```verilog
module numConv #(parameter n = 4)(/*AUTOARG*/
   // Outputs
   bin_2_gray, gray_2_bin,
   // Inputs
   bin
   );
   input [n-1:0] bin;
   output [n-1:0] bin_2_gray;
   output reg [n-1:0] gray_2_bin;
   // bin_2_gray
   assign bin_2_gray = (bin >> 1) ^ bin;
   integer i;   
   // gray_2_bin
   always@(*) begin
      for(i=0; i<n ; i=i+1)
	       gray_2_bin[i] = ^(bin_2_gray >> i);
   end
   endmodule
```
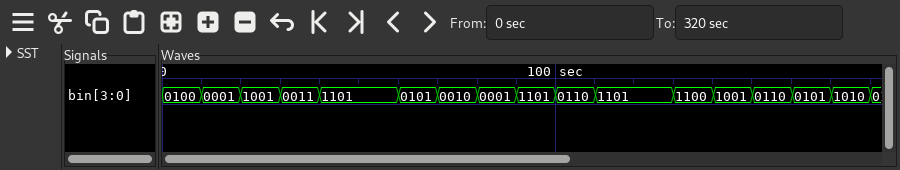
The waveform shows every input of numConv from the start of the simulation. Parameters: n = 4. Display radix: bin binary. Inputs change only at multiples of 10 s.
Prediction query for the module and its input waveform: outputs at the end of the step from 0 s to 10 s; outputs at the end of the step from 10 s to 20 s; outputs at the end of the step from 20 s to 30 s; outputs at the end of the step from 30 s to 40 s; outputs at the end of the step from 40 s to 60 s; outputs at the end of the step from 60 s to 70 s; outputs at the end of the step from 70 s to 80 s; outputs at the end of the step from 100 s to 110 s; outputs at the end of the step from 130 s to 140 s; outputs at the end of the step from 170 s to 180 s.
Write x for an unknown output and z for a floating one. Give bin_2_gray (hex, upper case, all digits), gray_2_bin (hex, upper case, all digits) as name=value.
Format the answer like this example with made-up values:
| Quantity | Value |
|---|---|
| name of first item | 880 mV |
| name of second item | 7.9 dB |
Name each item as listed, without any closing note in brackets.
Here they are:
| Quantity | Value |
|---|---|
| outputs at the end of the step from 0 s to 10 s | bin_2_gray=6, gray_2_bin=4 |
| outputs at the end of the step from 10 s to 20 s | bin_2_gray=1, gray_2_bin=1 |
| outputs at the end of the step from 20 s to 30 s | bin_2_gray=D, gray_2_bin=9 |
| outputs at the end of the step from 30 s to 40 s | bin_2_gray=2, gray_2_bin=3 |
| outputs at the end of the step from 40 s to 60 s | bin_2_gray=B, gray_2_bin=D |
| outputs at the end of the step from 60 s to 70 s | bin_2_gray=7, gray_2_bin=5 |
| outputs at the end of the step from 70 s to 80 s | bin_2_gray=3, gray_2_bin=2 |
| outputs at the end of the step from 100 s to 110 s | bin_2_gray=5, gray_2_bin=6 |
| outputs at the end of the step from 130 s to 140 s | bin_2_gray=A, gray_2_bin=C |
| outputs at the end of the step from 170 s to 180 s | bin_2_gray=F, gray_2_bin=A |
